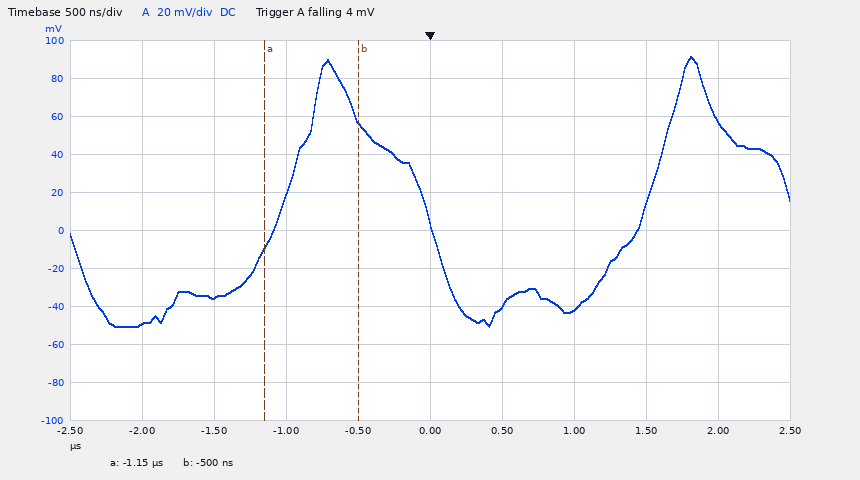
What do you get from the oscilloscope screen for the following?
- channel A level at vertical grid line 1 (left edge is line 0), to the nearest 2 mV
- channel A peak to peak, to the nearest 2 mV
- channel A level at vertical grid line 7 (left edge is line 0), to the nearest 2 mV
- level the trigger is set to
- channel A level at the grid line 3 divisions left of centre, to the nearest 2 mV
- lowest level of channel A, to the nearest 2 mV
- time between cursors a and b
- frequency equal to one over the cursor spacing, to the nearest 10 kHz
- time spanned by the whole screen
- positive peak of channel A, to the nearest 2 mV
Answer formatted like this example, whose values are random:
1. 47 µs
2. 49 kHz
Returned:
1. -50 mV
2. 142 mV
3. -42 mV
4. 4 mV
5. -36 mV
6. -50 mV
7. 650 ns
8. 1.54 MHz
9. 5 µs
10. 92 mV
